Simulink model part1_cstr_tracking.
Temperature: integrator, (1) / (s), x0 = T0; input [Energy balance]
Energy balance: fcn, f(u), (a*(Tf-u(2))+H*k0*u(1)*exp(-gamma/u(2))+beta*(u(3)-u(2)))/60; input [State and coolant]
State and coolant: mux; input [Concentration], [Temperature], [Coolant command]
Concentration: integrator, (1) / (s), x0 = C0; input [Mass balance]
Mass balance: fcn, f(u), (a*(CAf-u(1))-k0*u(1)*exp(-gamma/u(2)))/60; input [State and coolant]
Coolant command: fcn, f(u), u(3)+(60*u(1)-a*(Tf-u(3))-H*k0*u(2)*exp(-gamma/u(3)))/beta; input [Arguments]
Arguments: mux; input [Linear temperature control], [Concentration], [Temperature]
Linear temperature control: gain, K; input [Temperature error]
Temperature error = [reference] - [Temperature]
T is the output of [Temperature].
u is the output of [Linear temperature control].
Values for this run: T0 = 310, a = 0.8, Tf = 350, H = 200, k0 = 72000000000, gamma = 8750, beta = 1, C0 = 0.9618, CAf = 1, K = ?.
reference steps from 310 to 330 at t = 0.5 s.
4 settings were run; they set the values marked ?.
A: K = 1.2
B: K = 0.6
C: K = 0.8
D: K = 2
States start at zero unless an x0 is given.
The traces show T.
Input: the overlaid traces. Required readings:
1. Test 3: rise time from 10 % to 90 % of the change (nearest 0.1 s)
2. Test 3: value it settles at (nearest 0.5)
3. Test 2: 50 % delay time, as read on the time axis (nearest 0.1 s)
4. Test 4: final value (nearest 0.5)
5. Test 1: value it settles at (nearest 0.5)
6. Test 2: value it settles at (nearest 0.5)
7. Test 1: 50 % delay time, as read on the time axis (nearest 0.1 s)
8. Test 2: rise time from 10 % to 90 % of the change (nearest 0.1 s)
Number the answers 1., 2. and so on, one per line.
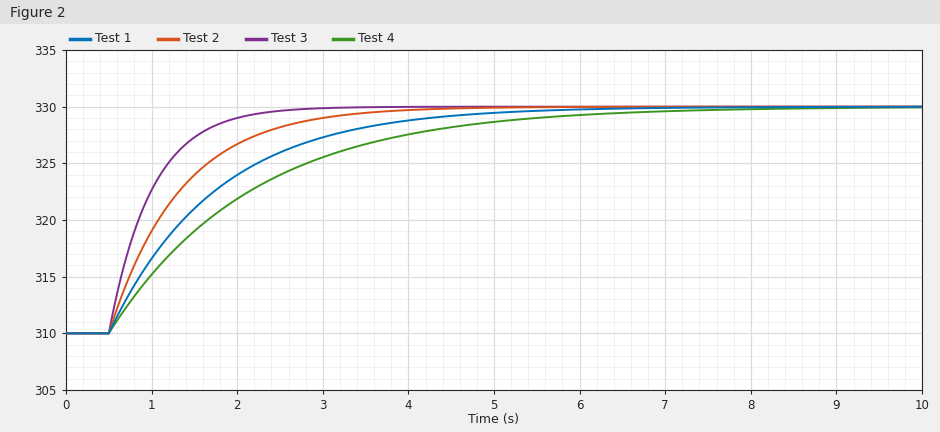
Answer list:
1. 1.1 s
2. 330.0
3. 1.1 s
4. 330.0
5. 330.0
6. 330.0
7. 1.4 s
8. 1.8 s
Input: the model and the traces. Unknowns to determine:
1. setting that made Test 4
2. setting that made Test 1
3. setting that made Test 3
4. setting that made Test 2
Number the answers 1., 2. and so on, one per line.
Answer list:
1. B
2. C
3. D
4. A
